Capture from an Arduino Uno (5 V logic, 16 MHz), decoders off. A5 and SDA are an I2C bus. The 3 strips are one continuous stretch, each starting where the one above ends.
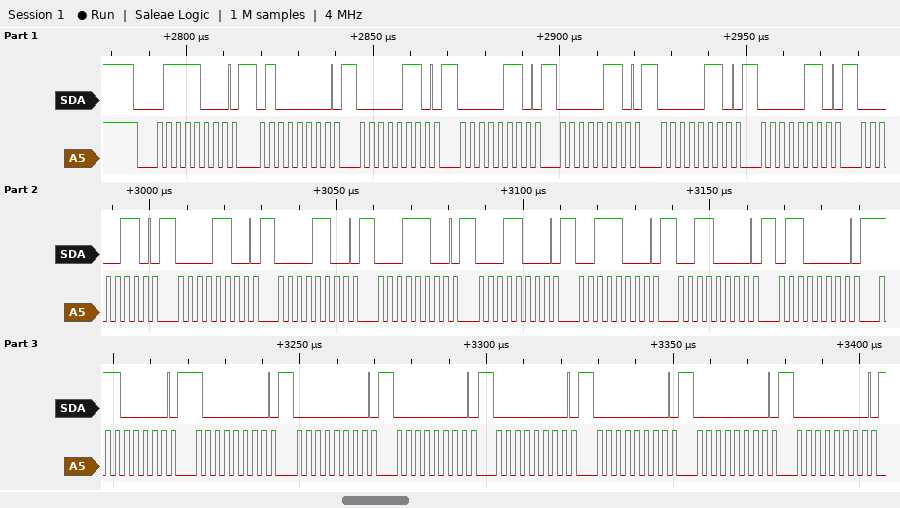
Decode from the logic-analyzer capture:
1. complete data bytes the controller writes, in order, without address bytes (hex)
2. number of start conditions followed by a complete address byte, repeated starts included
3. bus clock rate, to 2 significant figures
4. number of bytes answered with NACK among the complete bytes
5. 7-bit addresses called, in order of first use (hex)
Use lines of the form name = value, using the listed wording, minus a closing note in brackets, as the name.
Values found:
complete data bytes the controller writes, in order, without address bytes = 40 06 06 06 06 06 06 0C 0C 1C 18 38 30 60 E0 80 00 00 00 00 00 00
number of start conditions followed by a complete address byte, repeated starts included = 1
bus clock rate, to 2 significant figures = 400 kHz
number of bytes answered with NACK among the complete bytes = 0
7-bit addresses called, in order of first use = 0x3C
